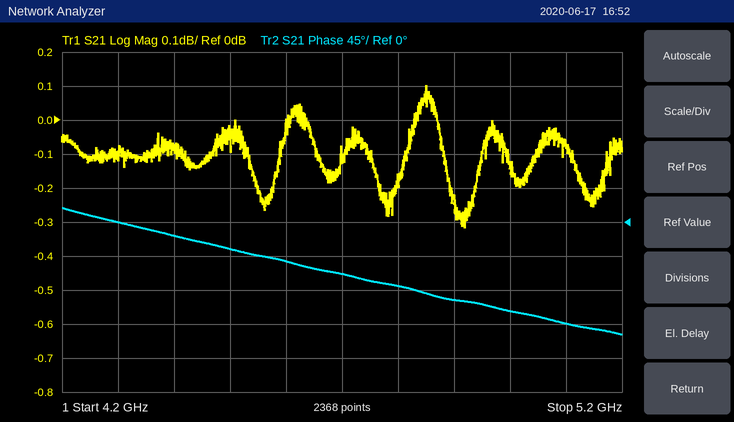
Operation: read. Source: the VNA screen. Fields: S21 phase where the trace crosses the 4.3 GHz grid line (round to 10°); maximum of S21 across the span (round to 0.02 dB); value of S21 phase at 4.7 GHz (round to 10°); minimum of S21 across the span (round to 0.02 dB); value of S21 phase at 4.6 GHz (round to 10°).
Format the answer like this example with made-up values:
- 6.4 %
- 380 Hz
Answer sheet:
- 0°
- 0.10 dB
- -70°
- -0.32 dB
- -50°
